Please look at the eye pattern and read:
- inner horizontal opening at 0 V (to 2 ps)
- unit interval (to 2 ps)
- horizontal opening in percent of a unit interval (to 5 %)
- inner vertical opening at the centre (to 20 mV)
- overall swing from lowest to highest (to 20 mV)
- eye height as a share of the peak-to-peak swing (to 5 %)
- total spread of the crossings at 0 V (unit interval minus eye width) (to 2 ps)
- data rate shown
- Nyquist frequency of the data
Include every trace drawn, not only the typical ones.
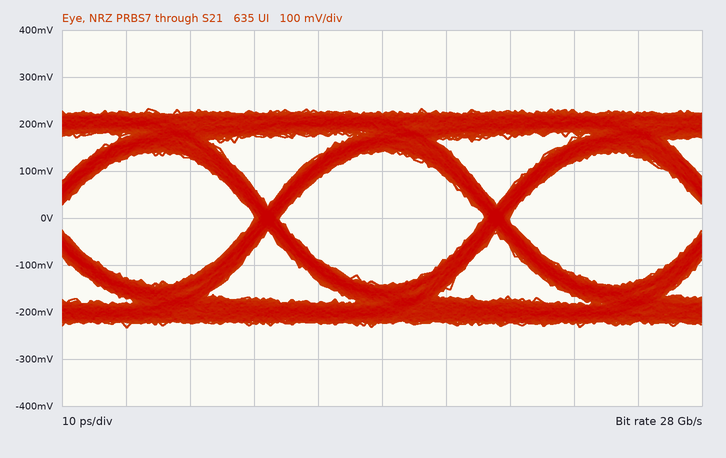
32 ps
36 ps
90 %
280 mV
460 mV
60 %
4 ps
28 Gb/s
14 GHz
